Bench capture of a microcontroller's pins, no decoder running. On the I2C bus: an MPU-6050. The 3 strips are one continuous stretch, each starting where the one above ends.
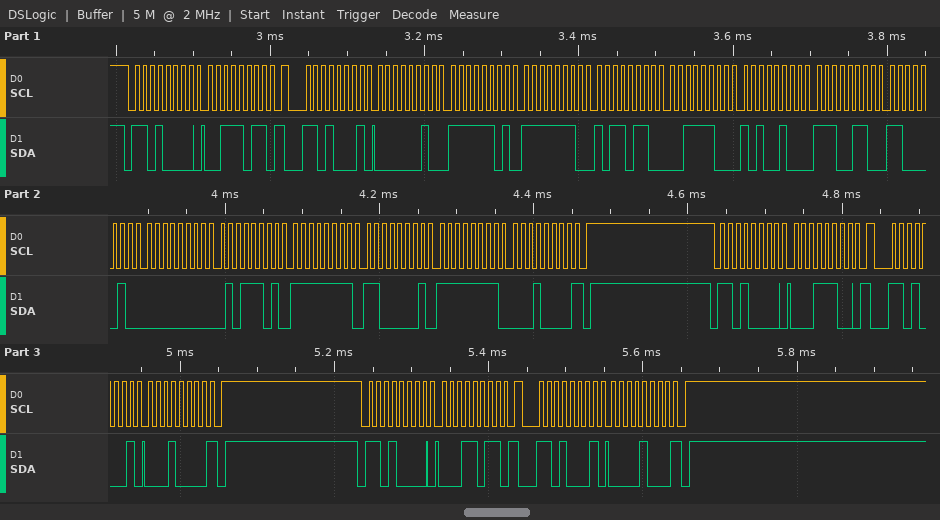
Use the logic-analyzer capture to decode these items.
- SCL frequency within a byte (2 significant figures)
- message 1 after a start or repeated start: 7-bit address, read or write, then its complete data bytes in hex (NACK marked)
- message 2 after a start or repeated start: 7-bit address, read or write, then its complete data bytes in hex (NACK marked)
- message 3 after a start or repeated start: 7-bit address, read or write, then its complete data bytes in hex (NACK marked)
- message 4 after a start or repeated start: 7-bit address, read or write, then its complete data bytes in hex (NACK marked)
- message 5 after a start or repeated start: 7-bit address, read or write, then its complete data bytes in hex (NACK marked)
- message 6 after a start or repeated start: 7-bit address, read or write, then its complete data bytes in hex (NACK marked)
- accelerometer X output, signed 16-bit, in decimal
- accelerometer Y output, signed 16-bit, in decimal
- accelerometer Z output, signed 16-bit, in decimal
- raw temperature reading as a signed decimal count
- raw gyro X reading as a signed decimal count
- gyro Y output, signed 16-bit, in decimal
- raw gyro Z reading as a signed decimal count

100 kHz
0x68 write: 3B
0x68 read: 02 FD FE B6 3C A4 E6 C2 00 5D FF C1 FF 10 NACK
0x68 write: 1C
0x68 read: 10 NACK
0x68 write: 1B
0x68 read: 08 NACK
765
-330
15524
-6462
93
-63
-240
